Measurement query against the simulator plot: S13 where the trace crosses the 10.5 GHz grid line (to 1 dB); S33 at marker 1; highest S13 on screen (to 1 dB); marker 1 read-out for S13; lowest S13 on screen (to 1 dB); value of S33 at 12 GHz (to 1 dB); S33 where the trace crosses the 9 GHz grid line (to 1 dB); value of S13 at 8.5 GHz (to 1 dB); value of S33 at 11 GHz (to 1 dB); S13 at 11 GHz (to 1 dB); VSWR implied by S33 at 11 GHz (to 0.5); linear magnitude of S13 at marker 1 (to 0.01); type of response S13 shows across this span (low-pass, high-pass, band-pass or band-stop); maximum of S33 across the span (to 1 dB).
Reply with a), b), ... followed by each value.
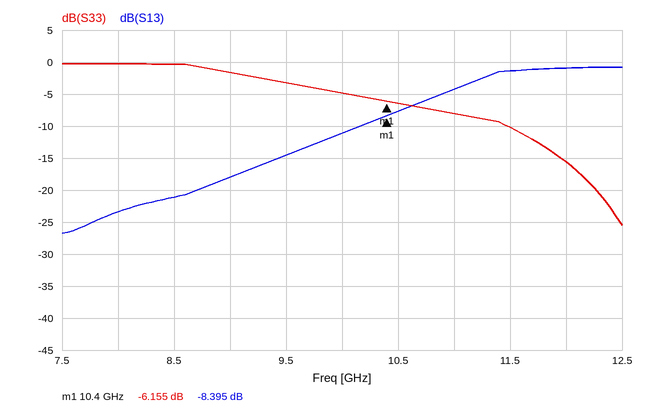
a) -8 dB
b) -6.155 dB
c) -1 dB
d) -8.395 dB
e) -27 dB
f) -16 dB
g) -2 dB
h) -21 dB
i) -8 dB
j) -4 dB
k) 2.5
l) 0.38
m) high-pass
n) 0 dB
